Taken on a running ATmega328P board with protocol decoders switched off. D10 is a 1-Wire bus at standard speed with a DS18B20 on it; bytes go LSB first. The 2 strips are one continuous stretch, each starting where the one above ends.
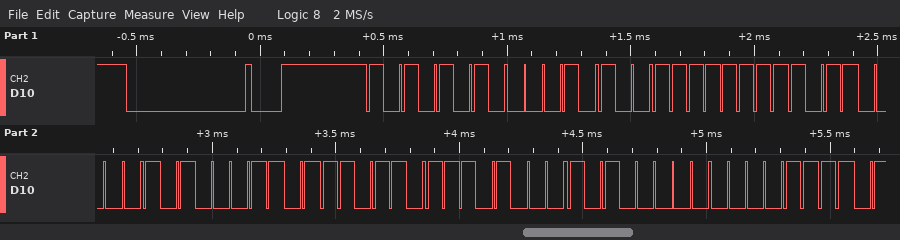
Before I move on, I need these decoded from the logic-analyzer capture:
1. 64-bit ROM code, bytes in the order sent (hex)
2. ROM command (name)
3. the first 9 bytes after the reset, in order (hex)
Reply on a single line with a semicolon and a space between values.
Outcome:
28 FF 0D C5 6E 17 05 F0; Match ROM; 55 28 FF 0D C5 6E 17 05 F0
